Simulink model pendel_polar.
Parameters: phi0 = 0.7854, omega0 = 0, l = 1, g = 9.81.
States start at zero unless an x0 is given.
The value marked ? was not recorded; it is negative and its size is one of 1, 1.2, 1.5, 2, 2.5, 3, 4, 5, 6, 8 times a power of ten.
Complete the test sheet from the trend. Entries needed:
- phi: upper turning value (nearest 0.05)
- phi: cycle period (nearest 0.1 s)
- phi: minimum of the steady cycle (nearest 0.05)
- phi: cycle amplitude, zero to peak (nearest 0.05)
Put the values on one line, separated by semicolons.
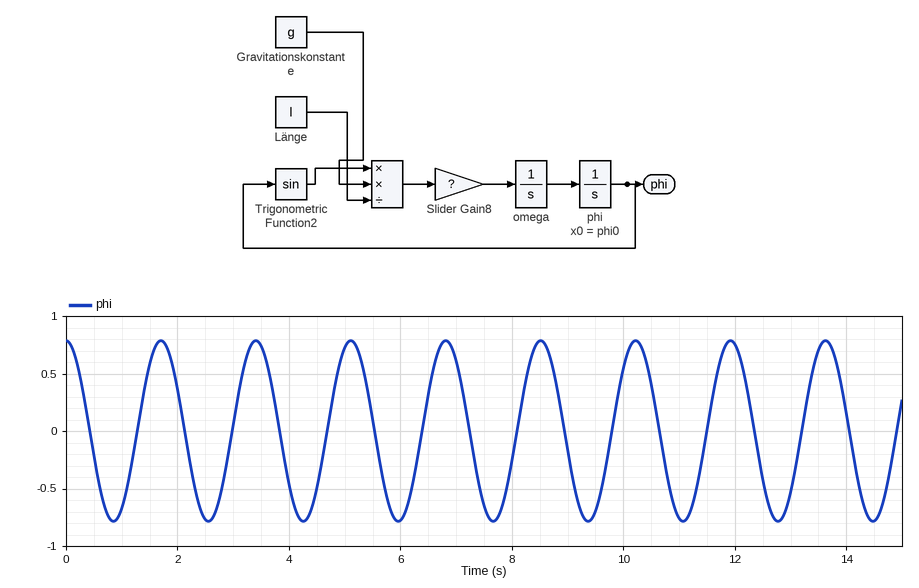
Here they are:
0.80; 1.7 s; -0.80; 0.80
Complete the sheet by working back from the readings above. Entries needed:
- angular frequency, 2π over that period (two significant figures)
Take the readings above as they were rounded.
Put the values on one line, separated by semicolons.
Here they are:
3.7 rad/s
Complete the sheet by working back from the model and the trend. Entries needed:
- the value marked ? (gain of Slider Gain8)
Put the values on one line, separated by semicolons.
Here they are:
-1.5
